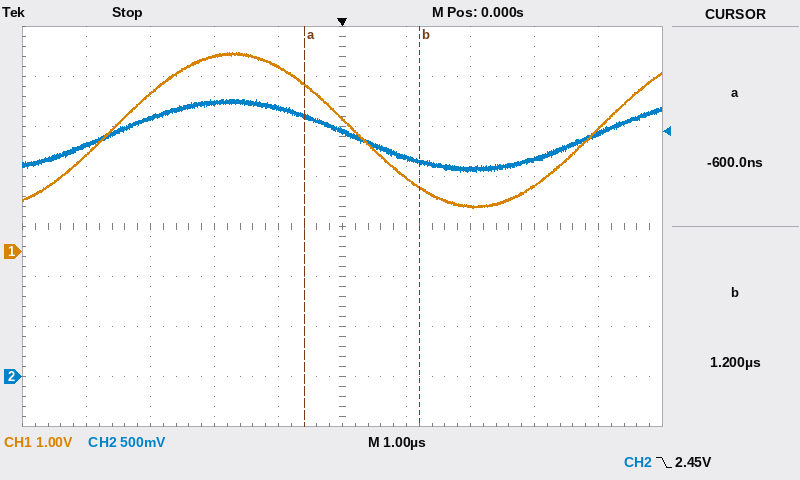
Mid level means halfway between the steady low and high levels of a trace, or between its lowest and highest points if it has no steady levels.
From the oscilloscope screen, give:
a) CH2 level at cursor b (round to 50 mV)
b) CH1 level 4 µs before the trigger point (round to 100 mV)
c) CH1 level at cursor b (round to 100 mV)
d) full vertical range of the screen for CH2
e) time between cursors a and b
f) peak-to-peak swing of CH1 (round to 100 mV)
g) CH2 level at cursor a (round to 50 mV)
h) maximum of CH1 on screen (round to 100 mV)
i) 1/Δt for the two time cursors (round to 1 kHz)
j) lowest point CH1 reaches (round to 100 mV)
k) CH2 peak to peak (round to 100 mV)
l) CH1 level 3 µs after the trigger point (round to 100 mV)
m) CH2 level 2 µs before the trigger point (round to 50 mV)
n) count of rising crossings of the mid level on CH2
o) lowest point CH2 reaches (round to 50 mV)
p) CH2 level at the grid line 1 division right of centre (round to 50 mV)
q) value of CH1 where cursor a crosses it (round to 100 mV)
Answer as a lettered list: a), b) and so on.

a) 2.15 V
b) 1.9 V
c) 1.3 V
d) 4 V
e) 1.8 µs
f) 3.1 V
g) 2.60 V
h) 4.0 V
i) 556 kHz
j) 900 mV
k) 700 mV
l) 1.3 V
m) 2.75 V
n) 2
o) 2.05 V
p) 2.20 V
q) 3.3 V
